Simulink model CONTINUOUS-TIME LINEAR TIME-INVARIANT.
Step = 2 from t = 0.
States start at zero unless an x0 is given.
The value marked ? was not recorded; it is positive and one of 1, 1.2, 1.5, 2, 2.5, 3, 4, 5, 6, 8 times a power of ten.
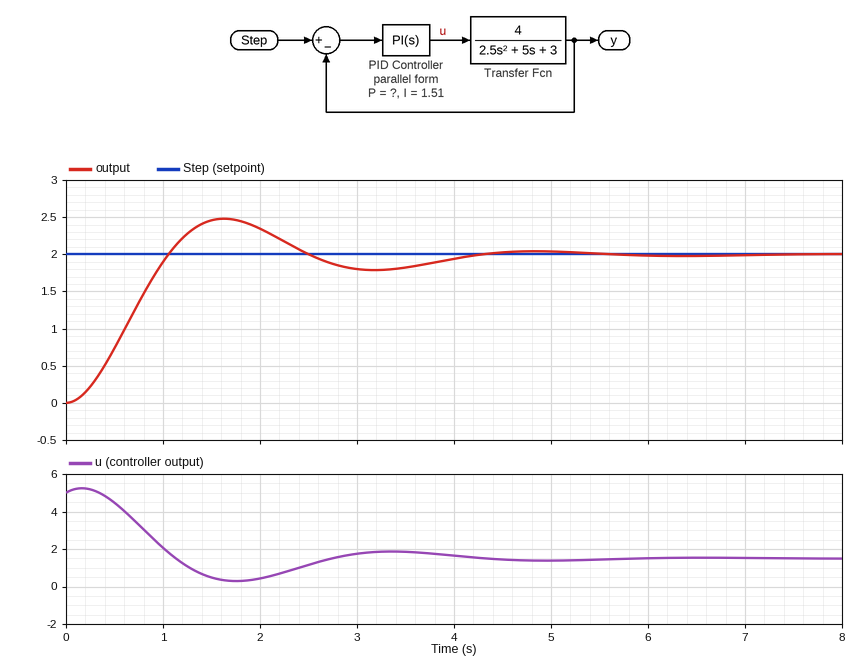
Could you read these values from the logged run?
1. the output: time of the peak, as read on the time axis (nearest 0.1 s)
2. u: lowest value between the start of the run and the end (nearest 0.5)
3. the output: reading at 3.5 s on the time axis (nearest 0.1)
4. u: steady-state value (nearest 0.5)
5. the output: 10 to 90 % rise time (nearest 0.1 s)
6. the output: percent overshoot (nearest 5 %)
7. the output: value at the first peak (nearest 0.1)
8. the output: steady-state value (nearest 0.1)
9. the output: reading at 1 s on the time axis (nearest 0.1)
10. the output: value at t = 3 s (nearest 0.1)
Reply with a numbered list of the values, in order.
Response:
1. 1.6 s
2. 0.5
3. 1.8
4. 1.5
5. 0.7 s
6. 25 %
7. 2.5
8. 2.0
9. 1.9
10. 1.8
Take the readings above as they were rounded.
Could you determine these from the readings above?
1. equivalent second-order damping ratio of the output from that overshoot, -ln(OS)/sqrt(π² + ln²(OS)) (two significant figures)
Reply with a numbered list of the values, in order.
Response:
1. 0.40
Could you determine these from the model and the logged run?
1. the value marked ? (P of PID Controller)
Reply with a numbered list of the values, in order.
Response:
1. 2.5
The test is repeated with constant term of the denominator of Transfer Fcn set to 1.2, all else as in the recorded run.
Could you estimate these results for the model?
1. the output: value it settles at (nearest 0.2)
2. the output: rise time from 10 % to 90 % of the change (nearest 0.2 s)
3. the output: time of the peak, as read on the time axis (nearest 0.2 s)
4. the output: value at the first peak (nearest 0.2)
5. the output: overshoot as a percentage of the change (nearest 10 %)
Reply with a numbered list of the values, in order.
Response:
1. 2.0
2. 0.6 s
3. 1.8 s
4. 2.8
5. 40 %
